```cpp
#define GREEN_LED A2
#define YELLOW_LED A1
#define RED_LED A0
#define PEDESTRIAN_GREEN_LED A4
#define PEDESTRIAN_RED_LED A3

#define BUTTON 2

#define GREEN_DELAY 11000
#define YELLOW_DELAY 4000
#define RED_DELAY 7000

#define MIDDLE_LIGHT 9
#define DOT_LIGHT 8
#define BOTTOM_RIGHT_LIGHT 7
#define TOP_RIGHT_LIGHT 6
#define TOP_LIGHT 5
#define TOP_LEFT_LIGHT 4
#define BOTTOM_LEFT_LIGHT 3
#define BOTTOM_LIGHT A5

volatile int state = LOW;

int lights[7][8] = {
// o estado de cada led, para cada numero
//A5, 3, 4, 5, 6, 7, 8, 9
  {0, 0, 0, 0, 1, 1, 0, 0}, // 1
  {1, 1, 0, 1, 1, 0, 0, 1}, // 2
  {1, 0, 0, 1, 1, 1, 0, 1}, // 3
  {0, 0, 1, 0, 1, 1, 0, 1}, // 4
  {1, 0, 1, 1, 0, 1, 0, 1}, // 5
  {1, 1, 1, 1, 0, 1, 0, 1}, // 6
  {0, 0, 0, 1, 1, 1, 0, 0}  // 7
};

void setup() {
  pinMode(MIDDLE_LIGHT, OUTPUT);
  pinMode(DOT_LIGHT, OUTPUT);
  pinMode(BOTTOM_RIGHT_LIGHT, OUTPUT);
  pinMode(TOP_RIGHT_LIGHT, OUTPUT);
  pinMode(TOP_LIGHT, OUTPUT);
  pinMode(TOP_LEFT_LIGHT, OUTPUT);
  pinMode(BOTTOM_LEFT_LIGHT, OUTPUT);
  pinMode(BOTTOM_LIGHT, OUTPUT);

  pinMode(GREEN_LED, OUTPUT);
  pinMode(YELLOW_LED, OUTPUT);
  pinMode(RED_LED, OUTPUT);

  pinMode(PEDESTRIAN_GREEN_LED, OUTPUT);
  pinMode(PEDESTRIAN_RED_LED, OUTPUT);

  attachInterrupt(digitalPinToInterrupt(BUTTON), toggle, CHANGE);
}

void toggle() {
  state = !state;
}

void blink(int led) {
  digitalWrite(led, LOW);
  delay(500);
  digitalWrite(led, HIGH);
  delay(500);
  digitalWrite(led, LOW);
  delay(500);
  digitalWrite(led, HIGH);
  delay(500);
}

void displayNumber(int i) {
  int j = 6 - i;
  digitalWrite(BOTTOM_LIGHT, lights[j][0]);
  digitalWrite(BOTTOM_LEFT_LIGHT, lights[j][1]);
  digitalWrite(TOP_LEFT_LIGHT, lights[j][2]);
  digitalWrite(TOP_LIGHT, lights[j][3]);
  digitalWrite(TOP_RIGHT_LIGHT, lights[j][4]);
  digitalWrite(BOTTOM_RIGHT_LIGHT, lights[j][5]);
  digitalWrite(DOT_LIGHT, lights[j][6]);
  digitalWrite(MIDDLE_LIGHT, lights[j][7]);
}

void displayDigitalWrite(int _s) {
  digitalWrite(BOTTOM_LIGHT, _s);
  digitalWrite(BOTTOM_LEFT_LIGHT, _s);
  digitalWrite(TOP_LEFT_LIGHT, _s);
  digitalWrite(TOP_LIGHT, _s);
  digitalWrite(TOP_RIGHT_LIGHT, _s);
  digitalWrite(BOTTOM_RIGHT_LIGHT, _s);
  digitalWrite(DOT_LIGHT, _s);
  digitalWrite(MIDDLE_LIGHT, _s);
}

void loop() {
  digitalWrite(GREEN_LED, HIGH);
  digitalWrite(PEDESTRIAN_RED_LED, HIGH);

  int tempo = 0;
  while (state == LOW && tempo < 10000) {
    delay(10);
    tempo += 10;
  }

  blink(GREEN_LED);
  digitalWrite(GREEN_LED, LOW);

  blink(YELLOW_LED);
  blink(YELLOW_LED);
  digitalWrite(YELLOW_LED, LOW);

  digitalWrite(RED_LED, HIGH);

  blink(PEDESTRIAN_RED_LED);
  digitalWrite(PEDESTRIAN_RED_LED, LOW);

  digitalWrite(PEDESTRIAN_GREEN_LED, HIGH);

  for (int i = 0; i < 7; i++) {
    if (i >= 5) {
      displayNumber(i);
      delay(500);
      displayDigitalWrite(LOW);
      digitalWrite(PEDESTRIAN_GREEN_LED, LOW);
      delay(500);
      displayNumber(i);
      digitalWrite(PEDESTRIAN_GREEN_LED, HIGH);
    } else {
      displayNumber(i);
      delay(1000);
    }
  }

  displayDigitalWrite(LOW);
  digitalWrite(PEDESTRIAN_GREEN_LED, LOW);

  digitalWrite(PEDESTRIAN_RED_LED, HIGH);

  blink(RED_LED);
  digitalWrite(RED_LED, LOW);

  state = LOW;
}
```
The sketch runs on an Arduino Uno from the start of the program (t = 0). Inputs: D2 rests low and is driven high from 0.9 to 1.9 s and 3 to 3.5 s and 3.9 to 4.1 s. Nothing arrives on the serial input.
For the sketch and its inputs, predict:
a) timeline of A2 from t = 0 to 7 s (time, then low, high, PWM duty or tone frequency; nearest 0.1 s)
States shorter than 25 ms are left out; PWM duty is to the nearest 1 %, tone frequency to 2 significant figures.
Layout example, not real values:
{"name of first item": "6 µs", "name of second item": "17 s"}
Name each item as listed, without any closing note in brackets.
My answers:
{"timeline of A2 from t = 0 to 7 s": "0 s high; 0.9 s low; 1.4 s high; 1.9 s low; 2.4 s high; 2.9 s low"}
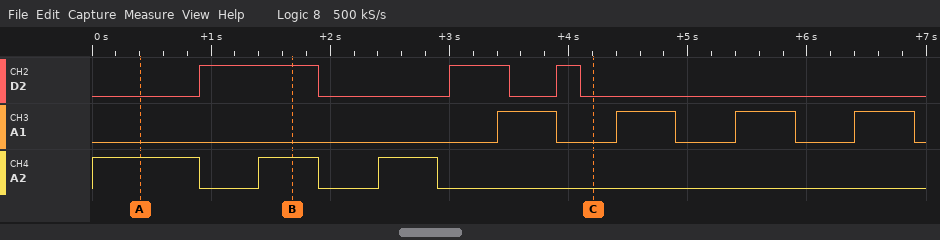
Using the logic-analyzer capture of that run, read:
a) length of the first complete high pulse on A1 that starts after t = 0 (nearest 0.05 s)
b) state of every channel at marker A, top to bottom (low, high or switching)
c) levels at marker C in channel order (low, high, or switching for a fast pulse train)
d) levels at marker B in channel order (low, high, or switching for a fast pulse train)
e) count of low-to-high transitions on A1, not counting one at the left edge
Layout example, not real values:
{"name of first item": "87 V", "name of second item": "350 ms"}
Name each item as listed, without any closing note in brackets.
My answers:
{"length of the first complete high pulse on A1 that starts after t = 0": "0.50 s", "state of every channel at marker A, top to bottom": "D2 low, A1 low, A2 high", "levels at marker C in channel order": "D2 low, A1 low, A2 low", "levels at marker B in channel order": "D2 high, A1 low, A2 high", "count of low-to-high transitions on A1, not counting one at the left edge": "4"}
